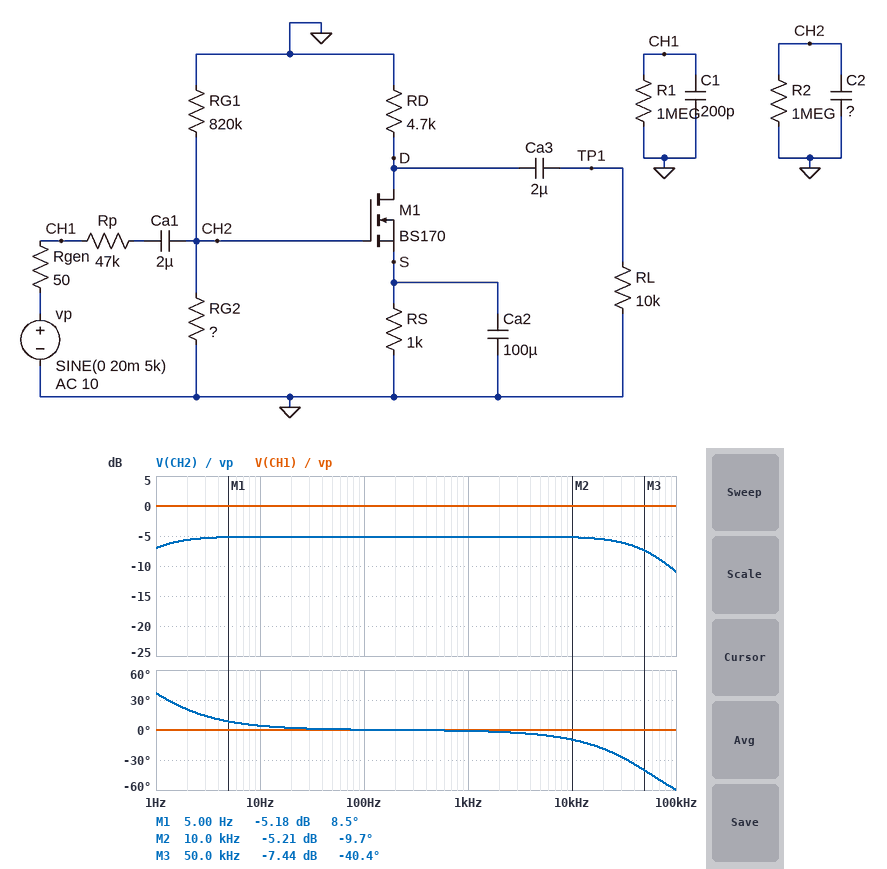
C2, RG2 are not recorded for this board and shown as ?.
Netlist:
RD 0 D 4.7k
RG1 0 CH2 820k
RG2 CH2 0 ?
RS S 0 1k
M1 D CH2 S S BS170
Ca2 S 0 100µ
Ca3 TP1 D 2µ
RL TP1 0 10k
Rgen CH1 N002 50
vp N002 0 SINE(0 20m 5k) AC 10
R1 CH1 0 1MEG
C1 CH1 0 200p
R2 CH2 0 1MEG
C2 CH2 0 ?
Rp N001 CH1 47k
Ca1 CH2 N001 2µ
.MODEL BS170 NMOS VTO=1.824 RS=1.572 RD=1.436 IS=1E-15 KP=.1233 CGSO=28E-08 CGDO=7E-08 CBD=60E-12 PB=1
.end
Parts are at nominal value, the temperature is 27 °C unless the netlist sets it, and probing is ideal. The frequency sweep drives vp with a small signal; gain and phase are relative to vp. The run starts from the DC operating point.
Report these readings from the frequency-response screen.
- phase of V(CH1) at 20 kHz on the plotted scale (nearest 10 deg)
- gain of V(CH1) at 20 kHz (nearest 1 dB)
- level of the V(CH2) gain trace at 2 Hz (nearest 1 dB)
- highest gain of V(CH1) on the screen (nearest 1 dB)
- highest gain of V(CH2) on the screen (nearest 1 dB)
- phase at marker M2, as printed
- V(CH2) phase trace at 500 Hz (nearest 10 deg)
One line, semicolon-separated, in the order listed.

0 deg; 0 dB; -6 dB; 0 dB; -5 dB; -9.7 deg; 0 deg
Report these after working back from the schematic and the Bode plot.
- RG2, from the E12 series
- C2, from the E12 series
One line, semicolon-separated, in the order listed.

68 kΩ; 68 pF
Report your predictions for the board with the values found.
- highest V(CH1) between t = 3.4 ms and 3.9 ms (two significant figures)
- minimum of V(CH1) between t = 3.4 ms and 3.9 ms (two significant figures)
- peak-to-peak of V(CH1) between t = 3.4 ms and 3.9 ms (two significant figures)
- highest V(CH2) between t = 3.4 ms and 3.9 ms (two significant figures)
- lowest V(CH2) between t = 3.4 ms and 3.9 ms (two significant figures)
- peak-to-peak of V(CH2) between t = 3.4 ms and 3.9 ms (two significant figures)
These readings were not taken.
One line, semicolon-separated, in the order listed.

20 mV; -20 mV; 40 mV; 11 mV; -11 mV; 22 mV
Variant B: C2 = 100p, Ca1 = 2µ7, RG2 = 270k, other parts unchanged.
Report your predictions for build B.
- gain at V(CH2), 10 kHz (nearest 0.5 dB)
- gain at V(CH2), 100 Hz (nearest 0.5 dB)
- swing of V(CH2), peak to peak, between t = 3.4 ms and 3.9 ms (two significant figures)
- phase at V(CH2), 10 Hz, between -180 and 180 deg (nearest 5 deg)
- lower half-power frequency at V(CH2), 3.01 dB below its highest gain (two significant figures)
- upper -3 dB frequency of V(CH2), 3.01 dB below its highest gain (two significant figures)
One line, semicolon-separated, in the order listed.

-2.5 dB; -2.0 dB; 31 mV; 0 deg; 270 mHz; 32 kHz
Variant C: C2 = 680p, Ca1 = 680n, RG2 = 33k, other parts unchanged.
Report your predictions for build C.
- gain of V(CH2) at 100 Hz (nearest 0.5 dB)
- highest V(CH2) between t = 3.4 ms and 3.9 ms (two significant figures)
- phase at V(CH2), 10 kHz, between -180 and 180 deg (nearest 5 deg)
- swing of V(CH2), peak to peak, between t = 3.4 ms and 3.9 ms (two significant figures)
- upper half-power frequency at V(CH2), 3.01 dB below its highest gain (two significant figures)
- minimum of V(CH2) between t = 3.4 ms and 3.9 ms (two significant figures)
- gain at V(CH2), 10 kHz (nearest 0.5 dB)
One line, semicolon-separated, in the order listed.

-8.0 dB; 7.3 mV; -40 deg; 15 mV; 12 kHz; -7.3 mV; -10.5 dB
